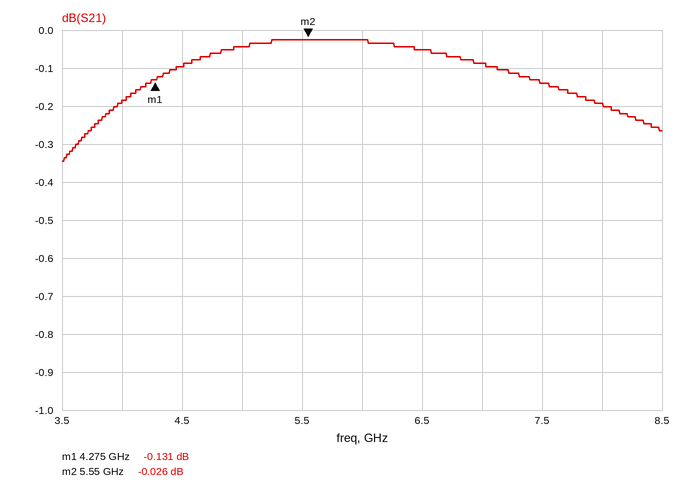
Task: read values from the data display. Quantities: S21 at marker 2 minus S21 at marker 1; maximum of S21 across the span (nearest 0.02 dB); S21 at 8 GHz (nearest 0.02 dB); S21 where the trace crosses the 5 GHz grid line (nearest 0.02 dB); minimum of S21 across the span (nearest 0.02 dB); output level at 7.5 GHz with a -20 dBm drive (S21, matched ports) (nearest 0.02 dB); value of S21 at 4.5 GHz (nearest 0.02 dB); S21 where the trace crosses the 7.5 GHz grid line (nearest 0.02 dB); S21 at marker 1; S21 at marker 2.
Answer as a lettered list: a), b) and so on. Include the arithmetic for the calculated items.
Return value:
a) -0.026 − (-0.131) = 0.105 dB
b) -0.02 dB
c) -0.20 dB
d) -0.04 dB
e) -0.34 dB
f) -20 dBm + (-0.14 dB) = -20.14 dBm
g) -0.10 dB
h) -0.14 dB
i) -0.131 dB
j) -0.026 dB
